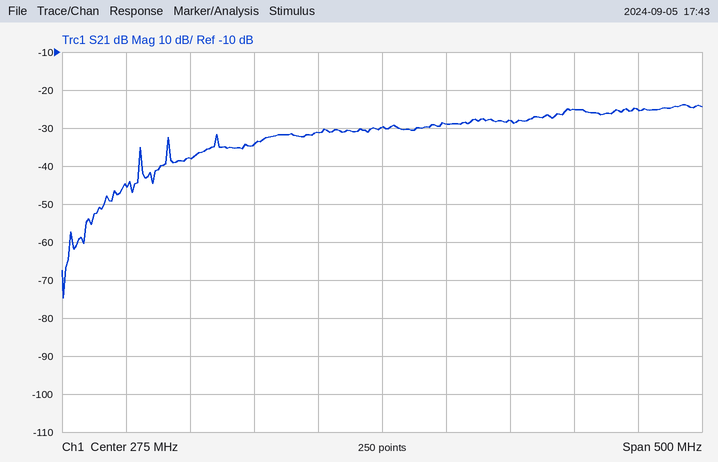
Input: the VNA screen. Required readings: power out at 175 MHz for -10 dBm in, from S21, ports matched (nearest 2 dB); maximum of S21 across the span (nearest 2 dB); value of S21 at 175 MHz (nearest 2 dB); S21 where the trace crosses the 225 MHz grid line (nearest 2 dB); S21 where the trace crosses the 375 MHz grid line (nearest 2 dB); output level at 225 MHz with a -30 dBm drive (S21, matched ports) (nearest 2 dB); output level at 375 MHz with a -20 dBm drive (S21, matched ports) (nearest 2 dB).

-44 dBm
-24 dB
-34 dB
-32 dB
-28 dB
-62 dBm
-48 dBm
